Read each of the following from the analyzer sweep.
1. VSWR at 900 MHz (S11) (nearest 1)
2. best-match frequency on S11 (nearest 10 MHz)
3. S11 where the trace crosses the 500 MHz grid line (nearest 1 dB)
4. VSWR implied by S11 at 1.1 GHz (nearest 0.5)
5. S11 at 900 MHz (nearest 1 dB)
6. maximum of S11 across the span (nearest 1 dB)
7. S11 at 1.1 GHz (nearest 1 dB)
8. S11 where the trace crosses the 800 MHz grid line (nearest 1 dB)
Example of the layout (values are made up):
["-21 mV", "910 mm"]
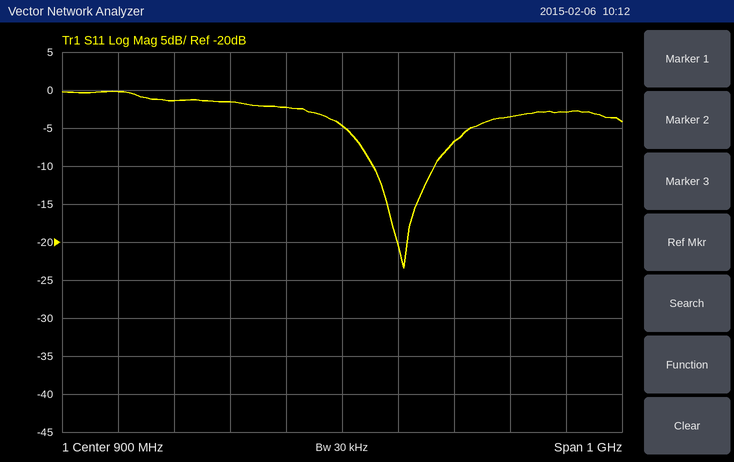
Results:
["4", "1.01 GHz", "0 dB", "2.5", "-5 dB", "0 dB", "-7 dB", "-2 dB"]
